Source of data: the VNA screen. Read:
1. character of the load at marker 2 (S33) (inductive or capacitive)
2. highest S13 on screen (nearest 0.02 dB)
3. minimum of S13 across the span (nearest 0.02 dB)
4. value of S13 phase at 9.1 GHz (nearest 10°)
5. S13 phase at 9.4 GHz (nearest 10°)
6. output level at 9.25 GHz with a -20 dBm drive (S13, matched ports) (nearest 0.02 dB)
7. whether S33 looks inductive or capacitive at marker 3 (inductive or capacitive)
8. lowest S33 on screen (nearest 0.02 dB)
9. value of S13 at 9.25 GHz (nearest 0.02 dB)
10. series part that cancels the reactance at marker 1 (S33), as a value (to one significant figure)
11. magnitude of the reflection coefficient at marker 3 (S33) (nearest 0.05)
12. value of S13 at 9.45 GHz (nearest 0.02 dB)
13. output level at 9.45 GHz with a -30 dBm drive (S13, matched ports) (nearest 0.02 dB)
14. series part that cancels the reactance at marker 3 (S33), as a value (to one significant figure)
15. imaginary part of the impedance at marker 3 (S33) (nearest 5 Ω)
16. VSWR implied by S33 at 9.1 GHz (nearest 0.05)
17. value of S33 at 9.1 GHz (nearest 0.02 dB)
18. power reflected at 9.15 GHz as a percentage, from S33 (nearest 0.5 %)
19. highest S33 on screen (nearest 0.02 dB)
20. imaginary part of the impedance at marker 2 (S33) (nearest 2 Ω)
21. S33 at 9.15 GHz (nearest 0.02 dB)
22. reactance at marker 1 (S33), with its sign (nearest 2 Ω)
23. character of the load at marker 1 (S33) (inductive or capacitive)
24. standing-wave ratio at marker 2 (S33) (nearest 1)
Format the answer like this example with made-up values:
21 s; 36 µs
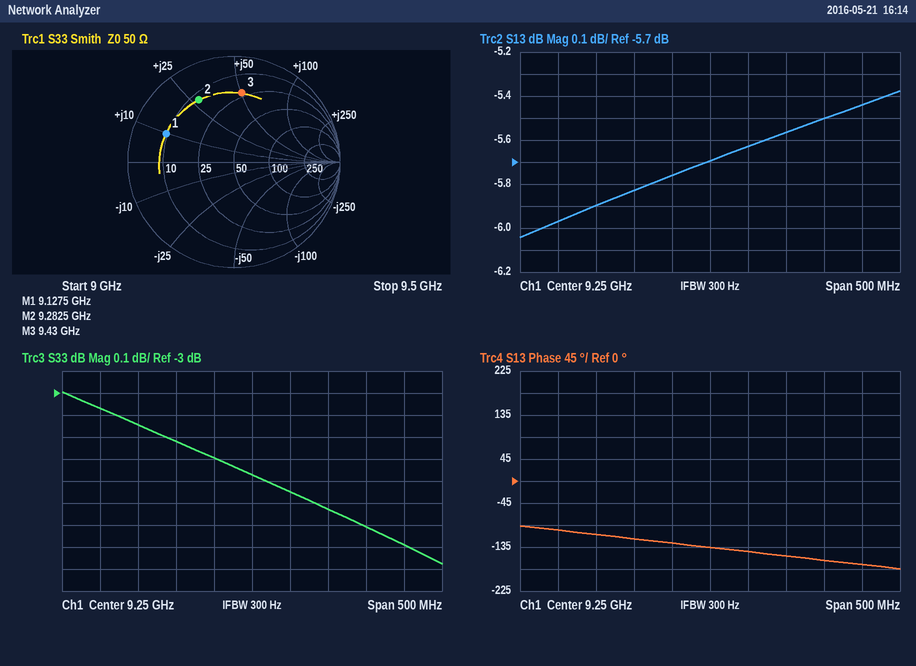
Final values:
inductive; -5.38 dB; -6.04 dB; -110°; -160°; -25.70 dBm; inductive; -3.78 dB; -5.70 dB; 2 pF; 0.65; -5.44 dB; -35.44 dBm; 300 fF; +50 Ω; 5.60; -3.14 dB; 47.5 %; -3.00 dB; +28 Ω; -3.22 dB; +10 Ω; inductive; 5
